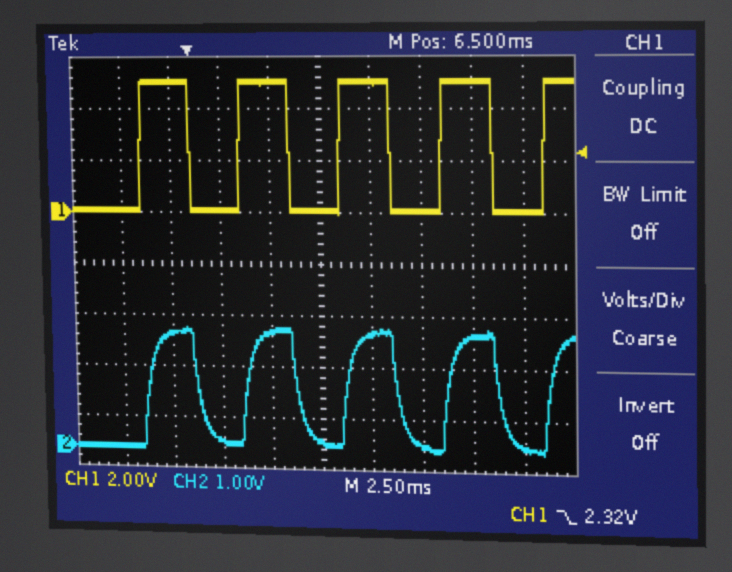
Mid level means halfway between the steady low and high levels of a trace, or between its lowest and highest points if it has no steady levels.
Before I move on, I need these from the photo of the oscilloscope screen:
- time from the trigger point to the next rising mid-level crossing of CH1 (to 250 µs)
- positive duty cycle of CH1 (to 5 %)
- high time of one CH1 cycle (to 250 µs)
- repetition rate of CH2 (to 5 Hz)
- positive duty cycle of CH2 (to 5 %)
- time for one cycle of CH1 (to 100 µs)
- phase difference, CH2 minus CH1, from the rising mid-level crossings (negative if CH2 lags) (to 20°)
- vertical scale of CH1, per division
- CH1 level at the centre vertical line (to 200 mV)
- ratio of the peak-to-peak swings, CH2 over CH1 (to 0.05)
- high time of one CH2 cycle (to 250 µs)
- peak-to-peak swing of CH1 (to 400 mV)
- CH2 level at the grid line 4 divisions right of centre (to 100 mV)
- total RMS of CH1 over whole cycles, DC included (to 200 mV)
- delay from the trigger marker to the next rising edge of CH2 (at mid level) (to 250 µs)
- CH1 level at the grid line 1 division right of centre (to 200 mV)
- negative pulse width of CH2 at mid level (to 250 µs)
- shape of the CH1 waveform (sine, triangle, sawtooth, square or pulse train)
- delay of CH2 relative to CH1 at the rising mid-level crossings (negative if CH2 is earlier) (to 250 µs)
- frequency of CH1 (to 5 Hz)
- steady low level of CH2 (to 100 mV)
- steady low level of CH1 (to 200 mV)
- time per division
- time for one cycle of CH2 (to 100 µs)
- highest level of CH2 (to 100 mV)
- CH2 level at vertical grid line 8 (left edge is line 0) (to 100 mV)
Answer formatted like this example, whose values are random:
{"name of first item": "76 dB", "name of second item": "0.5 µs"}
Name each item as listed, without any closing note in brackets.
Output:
{"time from the trigger point to the next rising mid-level crossing of CH1": "2.50 ms", "positive duty cycle of CH1": "50 %", "high time of one CH1 cycle": "2.50 ms", "repetition rate of CH2": "200 Hz", "positive duty cycle of CH2": "50 %", "time for one cycle of CH1": "5.0 ms", "phase difference, CH2 minus CH1, from the rising mid-level crossings (negative if CH2 lags)": "-20°", "vertical scale of CH1, per division": "2 V", "CH1 level at the centre vertical line": "0.0 V", "ratio of the peak-to-peak swings, CH2 over CH1": "0.45", "high time of one CH2 cycle": "2.50 ms", "peak-to-peak swing of CH1": "5.2 V", "CH2 level at the grid line 4 divisions right of centre": "100 mV", "total RMS of CH1 over whole cycles, DC included": "3.6 V", "delay from the trigger marker to the next rising edge of CH2 (at mid level)": "2.75 ms", "CH1 level at the grid line 1 division right of centre": "5.0 V", "negative pulse width of CH2 at mid level": "2.50 ms", "shape of the CH1 waveform": "square", "delay of CH2 relative to CH1 at the rising mid-level crossings (negative if CH2 is earlier)": "+250 µs", "frequency of CH1": "200 Hz", "steady low level of CH2": "0.0 V", "steady low level of CH1": "0.0 V", "time per division": "2.5 ms", "time for one cycle of CH2": "5.0 ms", "highest level of CH2": "2.4 V", "CH2 level at vertical grid line 8 (left edge is line 0)": "2.2 V"}
